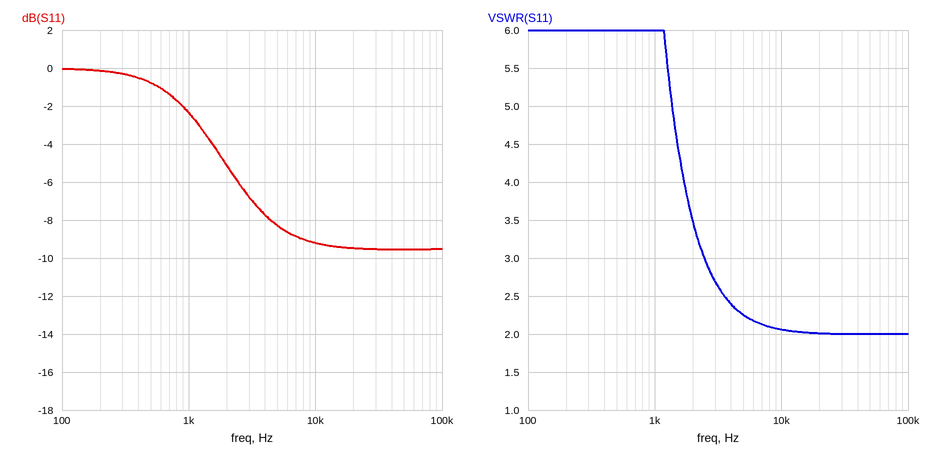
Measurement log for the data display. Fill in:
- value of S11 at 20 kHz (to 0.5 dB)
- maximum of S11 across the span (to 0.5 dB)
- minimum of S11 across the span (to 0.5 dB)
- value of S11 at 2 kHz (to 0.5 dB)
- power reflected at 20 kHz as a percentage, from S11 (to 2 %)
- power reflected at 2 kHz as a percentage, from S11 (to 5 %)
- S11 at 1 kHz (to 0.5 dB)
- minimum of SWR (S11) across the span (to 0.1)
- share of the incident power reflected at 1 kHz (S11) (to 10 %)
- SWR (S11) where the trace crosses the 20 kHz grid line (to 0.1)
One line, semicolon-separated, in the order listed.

-9.5 dB; 0.0 dB; -9.5 dB; -5.0 dB; 12 %; 30 %; -2.5 dB; 2.0; 60 %; 2.0
